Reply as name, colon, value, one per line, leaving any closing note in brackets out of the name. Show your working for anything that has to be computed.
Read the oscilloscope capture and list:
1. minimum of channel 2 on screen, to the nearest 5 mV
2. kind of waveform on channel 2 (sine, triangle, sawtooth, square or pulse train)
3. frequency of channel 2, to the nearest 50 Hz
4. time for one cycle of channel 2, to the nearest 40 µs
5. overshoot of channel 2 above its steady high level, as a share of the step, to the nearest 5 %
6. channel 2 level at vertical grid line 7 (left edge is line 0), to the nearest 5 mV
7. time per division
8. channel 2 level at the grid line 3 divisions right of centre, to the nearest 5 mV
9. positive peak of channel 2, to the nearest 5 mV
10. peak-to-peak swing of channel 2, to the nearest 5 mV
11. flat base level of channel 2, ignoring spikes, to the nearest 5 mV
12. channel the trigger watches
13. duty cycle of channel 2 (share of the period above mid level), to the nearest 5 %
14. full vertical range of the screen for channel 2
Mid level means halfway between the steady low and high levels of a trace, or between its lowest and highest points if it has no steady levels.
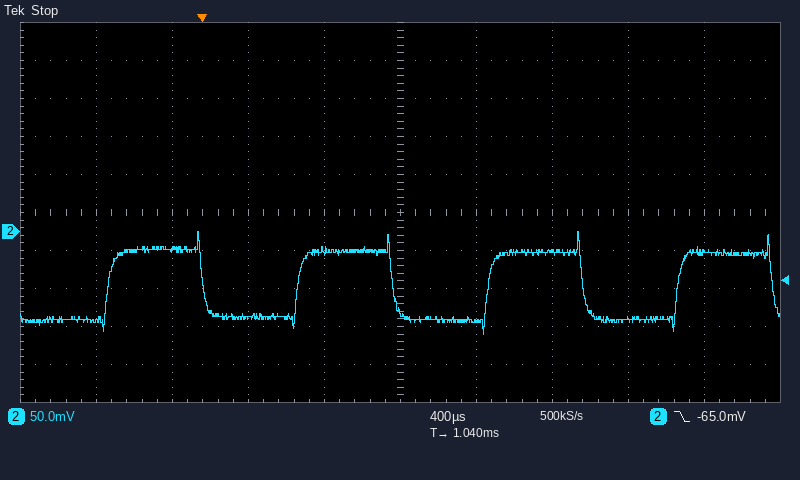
minimum of channel 2 on screen, to the nearest 5 mV: -135 mV
kind of waveform on channel 2: square
frequency of channel 2, to the nearest 50 Hz: 1 / 1.00 ms ≈ 1.00 kHz
time for one cycle of channel 2, to the nearest 40 µs: 1.00 ms
overshoot of channel 2 above its steady high level, as a share of the step, to the nearest 5 %: 30 %
channel 2 level at vertical grid line 7 (left edge is line 0), to the nearest 5 mV: -30 mV
time per division: 400 µs
channel 2 level at the grid line 3 divisions right of centre, to the nearest 5 mV: -115 mV
positive peak of channel 2, to the nearest 5 mV: 0 mV
peak-to-peak swing of channel 2, to the nearest 5 mV: 0 mV − (-135 mV) = 135 mV
flat base level of channel 2, ignoring spikes, to the nearest 5 mV: -115 mV
channel the trigger watches: channel 2
duty cycle of channel 2 (share of the period above mid level), to the nearest 5 %: 50 %
full vertical range of the screen for channel 2: 500 mV
